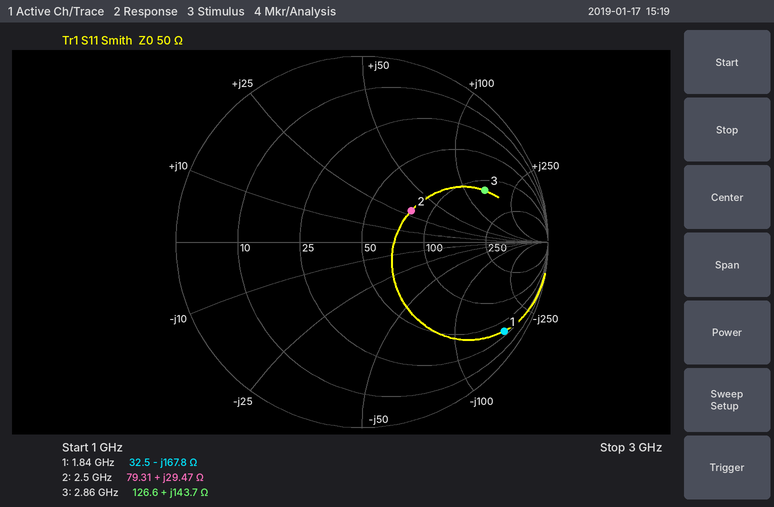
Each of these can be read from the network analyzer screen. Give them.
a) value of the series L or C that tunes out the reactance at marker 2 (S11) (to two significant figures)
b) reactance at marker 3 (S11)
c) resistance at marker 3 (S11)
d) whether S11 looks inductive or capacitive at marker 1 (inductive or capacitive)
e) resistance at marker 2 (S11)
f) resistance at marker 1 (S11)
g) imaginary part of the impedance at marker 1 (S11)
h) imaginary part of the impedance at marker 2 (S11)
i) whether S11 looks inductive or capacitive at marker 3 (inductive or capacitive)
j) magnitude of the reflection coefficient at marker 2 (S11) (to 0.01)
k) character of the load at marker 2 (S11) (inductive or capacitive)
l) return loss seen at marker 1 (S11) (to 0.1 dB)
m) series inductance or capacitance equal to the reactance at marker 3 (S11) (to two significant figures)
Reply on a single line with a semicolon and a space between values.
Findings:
2.2 pF; +143.7 Ω; 126.6 Ω; capacitive; 79.31 Ω; 32.5 Ω; -167.8 Ω; +29.47 Ω; inductive; 0.31; inductive; 0.9 dB; 8.0 nH
